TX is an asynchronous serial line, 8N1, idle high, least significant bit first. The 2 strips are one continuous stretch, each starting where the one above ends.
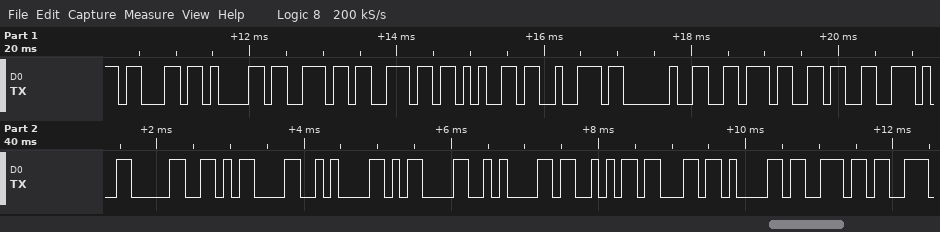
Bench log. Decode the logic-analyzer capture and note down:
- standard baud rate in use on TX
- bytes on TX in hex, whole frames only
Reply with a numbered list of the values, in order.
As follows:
1. 9600 baud
2. 63 61 6E 6E 65 72 20 76 36 2E 30 0D 0A 0D 0A 53 63 61 6E
